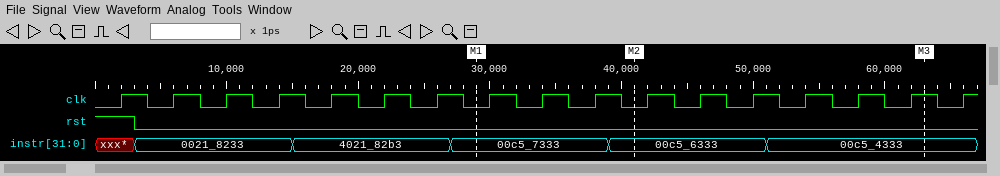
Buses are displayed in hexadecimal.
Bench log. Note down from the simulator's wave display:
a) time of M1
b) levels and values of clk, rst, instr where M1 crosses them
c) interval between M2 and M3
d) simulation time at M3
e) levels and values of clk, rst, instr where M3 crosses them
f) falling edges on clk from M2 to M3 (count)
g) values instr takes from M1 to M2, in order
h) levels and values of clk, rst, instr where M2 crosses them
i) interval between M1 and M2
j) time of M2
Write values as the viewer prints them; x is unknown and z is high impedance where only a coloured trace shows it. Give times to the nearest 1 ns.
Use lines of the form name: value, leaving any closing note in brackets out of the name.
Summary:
time of M1: 29 ns
levels and values of clk, rst, instr where M1 crosses them: clk=0, rst=0, instr=00c5_7333
interval between M2 and M3: 22 ns
simulation time at M3: 63 ns
levels and values of clk, rst, instr where M3 crosses them: clk=1, rst=0, instr=00c5_4333
falling edges on clk from M2 to M3: 5
values instr takes from M1 to M2, in order: 00c5_7333, 00c5_6333
levels and values of clk, rst, instr where M2 crosses them: clk=0, rst=0, instr=00c5_6333
interval between M1 and M2: 12 ns
time of M2: 41 ns
